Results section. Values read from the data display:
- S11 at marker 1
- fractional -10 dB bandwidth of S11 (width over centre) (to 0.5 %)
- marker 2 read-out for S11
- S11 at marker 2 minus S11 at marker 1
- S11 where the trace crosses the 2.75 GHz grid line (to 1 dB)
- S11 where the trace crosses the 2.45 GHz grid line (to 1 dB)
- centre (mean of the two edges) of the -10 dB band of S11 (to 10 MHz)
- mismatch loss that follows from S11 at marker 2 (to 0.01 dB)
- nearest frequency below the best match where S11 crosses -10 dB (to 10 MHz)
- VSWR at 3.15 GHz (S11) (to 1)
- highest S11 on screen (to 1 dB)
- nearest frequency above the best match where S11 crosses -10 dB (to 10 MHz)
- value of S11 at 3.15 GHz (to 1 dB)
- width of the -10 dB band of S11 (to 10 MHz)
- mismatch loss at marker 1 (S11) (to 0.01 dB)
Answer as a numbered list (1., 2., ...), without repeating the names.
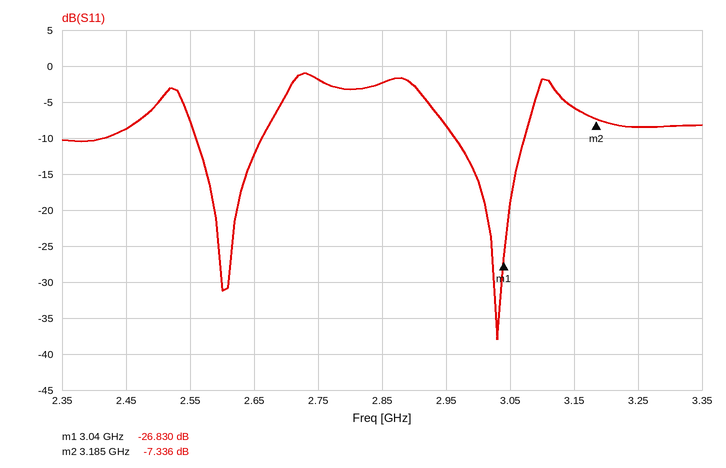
1. -26.830 dB
2. 3.5 %
3. -7.336 dB
4. 19.494 dB
5. -2 dB
6. -9 dB
7. 3.02 GHz
8. 0.89 dB
9. 2.96 GHz
10. 3
11. -1 dB
12. 3.07 GHz
13. -6 dB
14. 110 MHz
15. 0.01 dB
